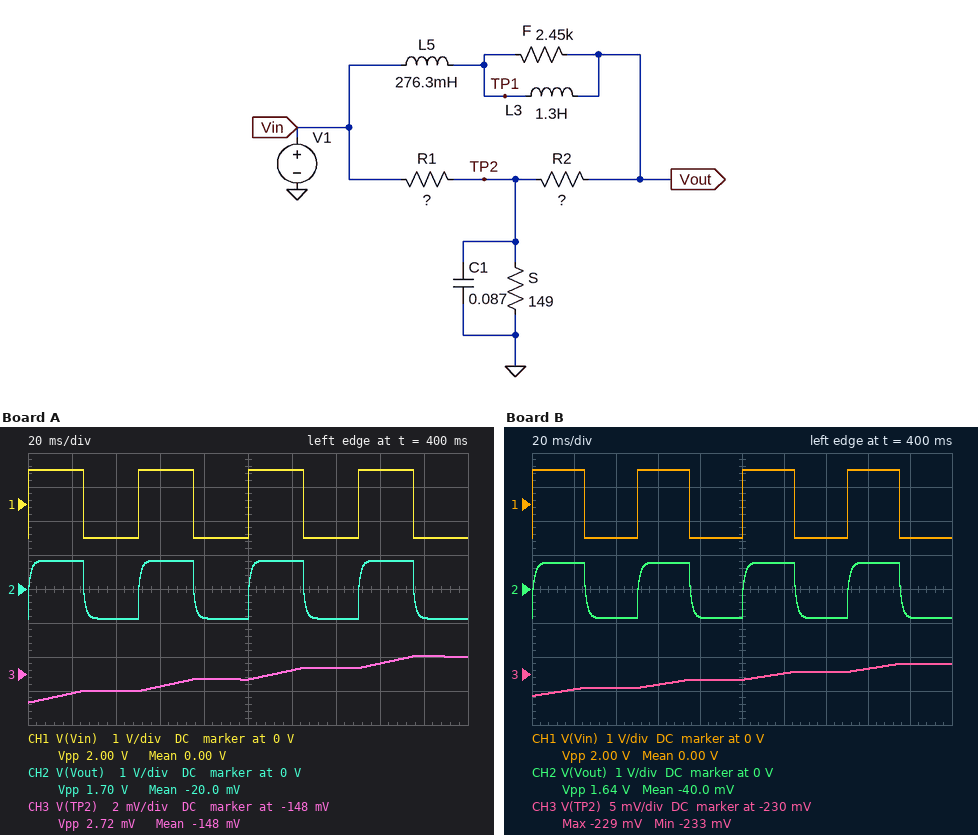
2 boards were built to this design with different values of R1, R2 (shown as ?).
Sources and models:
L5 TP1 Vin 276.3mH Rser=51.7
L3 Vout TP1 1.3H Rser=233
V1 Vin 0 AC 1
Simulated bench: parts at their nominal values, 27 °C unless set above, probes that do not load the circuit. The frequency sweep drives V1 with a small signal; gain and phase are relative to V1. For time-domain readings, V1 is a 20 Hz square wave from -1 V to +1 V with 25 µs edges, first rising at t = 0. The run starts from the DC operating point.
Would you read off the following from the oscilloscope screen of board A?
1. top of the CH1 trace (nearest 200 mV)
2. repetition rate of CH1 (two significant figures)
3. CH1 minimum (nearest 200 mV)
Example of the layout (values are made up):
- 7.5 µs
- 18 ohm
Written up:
- 1.0 V
- 20 Hz
- -1.0 V
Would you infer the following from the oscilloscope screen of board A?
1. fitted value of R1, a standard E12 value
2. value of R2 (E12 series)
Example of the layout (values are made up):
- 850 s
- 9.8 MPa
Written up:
- 1.5 kΩ
- 1.5 kΩ
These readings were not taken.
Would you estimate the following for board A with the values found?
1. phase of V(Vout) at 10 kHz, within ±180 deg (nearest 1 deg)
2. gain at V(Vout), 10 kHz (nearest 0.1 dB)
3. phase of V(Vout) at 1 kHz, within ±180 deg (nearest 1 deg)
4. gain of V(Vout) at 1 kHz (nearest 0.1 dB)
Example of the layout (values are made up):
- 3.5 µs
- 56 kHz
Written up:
- -77 deg
- -21.5 dB
- -32 deg
- -9.5 dB
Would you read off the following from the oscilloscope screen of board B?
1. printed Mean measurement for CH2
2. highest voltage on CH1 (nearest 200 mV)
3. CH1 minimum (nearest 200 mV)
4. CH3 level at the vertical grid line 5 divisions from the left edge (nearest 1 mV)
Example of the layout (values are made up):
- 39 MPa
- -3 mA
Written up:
- -40.0 mV
- 1.0 V
- -1.0 V
- -231 mV
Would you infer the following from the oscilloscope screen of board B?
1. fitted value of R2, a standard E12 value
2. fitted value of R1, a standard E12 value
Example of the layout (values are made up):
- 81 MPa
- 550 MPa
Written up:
- 1.2 kΩ
- 680 Ω
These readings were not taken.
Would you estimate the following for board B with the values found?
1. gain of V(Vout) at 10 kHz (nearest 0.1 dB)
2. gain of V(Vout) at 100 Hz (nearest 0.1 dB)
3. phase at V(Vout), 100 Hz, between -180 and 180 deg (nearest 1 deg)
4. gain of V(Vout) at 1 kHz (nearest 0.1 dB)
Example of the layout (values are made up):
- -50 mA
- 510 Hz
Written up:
- -23.4 dB
- -3.7 dB
- -26 deg
- -10.9 dB
